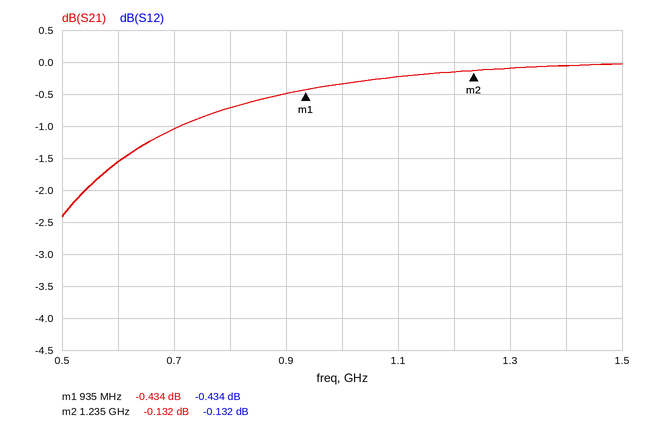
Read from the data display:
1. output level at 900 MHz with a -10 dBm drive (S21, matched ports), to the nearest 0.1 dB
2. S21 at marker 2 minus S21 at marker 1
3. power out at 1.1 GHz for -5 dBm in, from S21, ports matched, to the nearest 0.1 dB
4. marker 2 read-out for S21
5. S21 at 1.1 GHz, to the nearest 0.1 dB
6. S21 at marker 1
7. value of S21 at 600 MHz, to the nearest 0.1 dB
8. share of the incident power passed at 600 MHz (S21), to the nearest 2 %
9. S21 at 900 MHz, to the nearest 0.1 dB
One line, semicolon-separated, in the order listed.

-10.5 dBm; 0.302 dB; -5.2 dBm; -0.132 dB; -0.2 dB; -0.434 dB; -1.6 dB; 70 %; -0.5 dB
